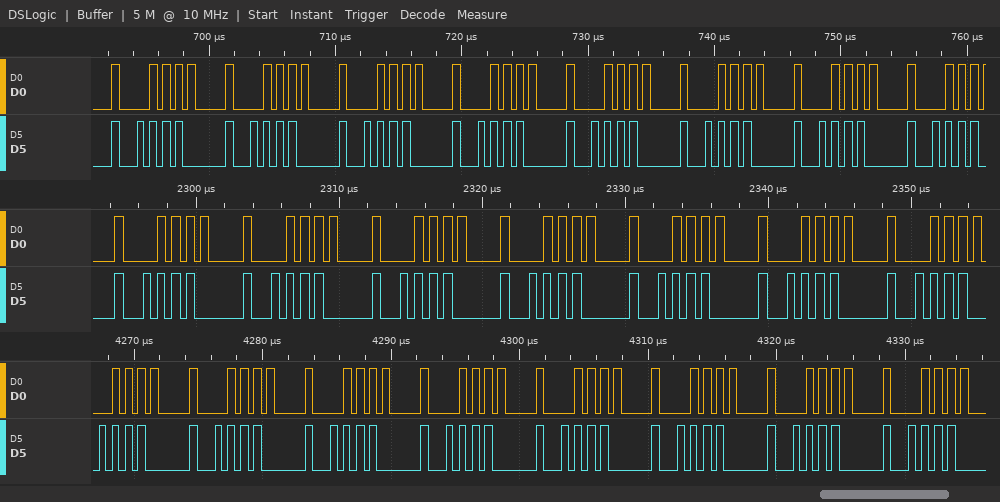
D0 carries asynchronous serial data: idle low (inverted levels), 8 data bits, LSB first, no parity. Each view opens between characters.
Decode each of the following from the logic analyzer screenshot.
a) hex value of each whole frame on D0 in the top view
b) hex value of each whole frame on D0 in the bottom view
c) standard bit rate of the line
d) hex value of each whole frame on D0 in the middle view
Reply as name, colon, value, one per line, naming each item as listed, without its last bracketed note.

hex value of each whole frame on D0 in the top view: 5F, 7D, D5, 5F, 7D, D5, 5F, 7D, D5, 5F, 7D
hex value of each whole frame on D0 in the bottom view: D5, 5F, 7D, D5, 5F, 7D, D5, 5F, 7D, D5, 5F
standard bit rate of the line: 2000000 baud
hex value of each whole frame on D0 in the middle view: 5F, 7D, D5, 5F, 7D, D5, 5F, 7D, D5, 5F
